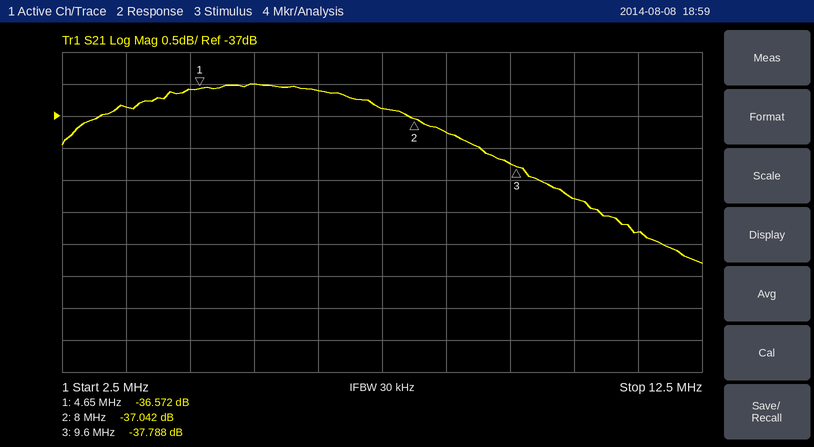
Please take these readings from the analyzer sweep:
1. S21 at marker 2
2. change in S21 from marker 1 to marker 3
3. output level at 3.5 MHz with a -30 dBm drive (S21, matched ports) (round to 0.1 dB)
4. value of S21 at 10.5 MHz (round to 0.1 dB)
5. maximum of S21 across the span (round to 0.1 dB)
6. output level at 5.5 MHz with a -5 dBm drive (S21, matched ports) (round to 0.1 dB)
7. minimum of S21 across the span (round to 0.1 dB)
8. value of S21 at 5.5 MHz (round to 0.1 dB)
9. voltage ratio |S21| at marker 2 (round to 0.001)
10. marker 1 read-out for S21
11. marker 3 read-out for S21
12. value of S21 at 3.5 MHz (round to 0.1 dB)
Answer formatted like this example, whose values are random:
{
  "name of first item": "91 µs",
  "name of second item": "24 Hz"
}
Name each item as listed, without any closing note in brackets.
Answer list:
{
  "S21 at marker 2": "-37.042 dB",
  "change in S21 from marker 1 to marker 3": "-1.216 dB",
  "output level at 3.5 MHz with a -30 dBm drive (S21, matched ports)": "-66.9 dBm",
  "value of S21 at 10.5 MHz": "-38.3 dB",
  "maximum of S21 across the span": "-36.5 dB",
  "output level at 5.5 MHz with a -5 dBm drive (S21, matched ports)": "-41.5 dBm",
  "minimum of S21 across the span": "-39.3 dB",
  "value of S21 at 5.5 MHz": "-36.5 dB",
  "voltage ratio |S21| at marker 2": "0.014",
  "marker 1 read-out for S21": "-36.572 dB",
  "marker 3 read-out for S21": "-37.788 dB",
  "value of S21 at 3.5 MHz": "-36.9 dB"
}
